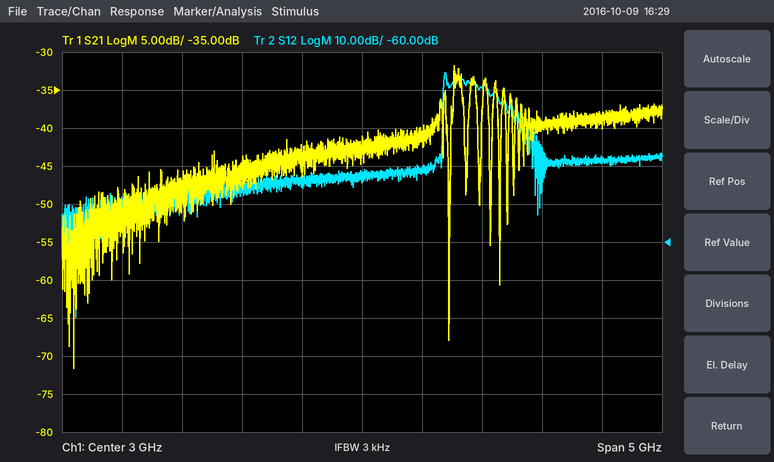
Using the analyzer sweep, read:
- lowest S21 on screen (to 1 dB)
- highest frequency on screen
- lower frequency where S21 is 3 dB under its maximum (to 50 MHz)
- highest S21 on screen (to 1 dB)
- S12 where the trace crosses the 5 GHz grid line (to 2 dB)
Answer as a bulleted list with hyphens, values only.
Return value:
- -72 dB
- 5.5 GHz
- 3.75 GHz
- -32 dB
- -38 dB
